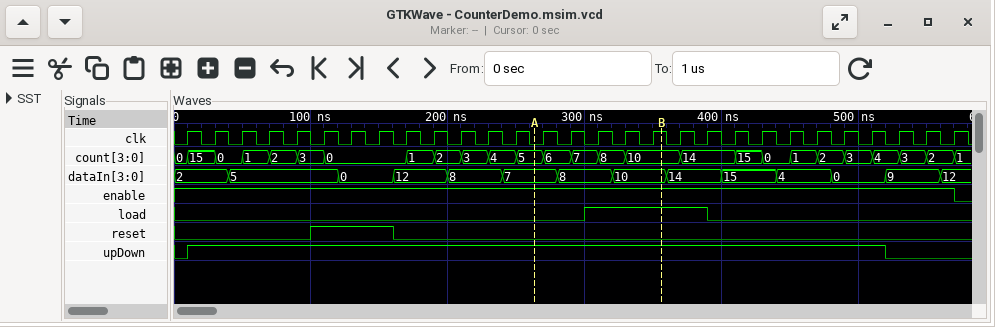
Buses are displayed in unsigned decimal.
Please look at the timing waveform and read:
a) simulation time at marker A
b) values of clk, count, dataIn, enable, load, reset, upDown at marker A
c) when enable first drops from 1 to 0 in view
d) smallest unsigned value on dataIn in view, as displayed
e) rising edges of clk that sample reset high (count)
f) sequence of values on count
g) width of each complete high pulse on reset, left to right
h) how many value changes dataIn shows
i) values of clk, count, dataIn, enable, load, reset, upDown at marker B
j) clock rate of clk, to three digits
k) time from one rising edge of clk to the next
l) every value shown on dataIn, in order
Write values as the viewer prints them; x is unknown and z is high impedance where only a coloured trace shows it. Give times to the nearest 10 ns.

260 ns
clk=0, count=5, dataIn=7, enable=1, load=0, reset=0, upDown=1
570 ns
0
3
0, 15, 0, 1, 2, 3, 0, 1, 2, 3, 4, 5, 6, 7, 8, 10, 14, 15, 0, 1, 2, 3, 4, 3, 2, 1
60 ns
13
clk=1, count=10, dataIn=10, enable=1, load=1, reset=0, upDown=1
50.0 MHz
20 ns
2, 5, 0, 12, 8, 7, 8, 10, 14, 15, 4, 0, 9, 12
